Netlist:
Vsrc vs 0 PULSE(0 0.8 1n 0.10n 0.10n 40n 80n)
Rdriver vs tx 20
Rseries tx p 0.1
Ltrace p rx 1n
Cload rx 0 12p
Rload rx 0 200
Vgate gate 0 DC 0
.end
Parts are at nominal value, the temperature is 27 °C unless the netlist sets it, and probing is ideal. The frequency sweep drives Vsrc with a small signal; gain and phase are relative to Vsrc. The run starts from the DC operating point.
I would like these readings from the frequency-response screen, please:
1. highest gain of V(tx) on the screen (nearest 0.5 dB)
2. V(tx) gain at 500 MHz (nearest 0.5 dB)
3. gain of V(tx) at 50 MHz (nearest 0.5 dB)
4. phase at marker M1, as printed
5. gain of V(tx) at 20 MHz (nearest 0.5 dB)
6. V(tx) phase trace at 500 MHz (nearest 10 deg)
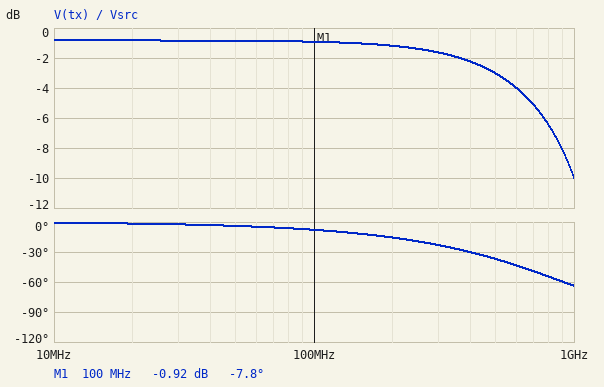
-1.0 dB
-3.0 dB
-1.0 dB
-7.8 deg
-1.0 dB
-40 deg
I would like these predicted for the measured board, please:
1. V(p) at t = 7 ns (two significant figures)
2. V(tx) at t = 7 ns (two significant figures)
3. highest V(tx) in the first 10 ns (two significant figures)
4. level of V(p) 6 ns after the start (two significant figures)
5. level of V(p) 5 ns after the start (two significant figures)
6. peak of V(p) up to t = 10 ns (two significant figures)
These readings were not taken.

730 mV
730 mV
730 mV
730 mV
730 mV
730 mV
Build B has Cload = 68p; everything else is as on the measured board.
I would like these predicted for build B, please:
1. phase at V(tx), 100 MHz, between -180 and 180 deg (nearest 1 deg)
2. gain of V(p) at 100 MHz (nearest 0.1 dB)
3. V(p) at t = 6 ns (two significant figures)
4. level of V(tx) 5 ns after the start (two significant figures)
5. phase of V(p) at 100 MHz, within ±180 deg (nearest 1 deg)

-38 deg
-3.0 dB
710 mV
700 mV
-39 deg
